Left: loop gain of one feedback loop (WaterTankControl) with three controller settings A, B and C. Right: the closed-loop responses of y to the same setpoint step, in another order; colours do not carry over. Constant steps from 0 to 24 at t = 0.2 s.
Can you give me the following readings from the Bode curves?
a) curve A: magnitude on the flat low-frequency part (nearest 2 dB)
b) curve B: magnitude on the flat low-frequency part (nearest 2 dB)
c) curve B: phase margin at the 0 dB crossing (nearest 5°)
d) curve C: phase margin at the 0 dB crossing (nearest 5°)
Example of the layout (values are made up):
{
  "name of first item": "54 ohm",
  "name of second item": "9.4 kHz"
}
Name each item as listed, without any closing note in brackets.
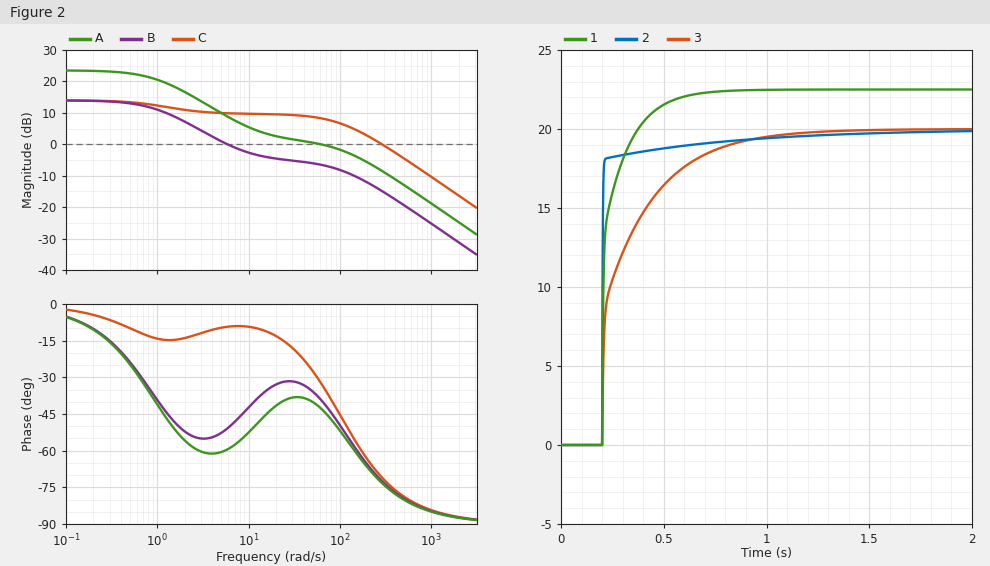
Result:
{
  "curve A: magnitude on the flat low-frequency part": "24 dB",
  "curve B: magnitude on the flat low-frequency part": "14 dB",
  "curve B: phase margin at the 0 dB crossing": "130°",
  "curve C: phase margin at the 0 dB crossing": "110°"
}
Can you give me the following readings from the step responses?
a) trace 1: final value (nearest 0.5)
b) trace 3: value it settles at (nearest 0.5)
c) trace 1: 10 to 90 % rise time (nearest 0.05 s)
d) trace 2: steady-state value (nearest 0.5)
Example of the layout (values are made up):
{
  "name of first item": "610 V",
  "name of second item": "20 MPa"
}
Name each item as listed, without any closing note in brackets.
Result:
{
  "trace 1: final value": "22.5",
  "trace 3: value it settles at": "20.0",
  "trace 1: 10 to 90 % rise time": "0.20 s",
  "trace 2: steady-state value": "20.0"
}
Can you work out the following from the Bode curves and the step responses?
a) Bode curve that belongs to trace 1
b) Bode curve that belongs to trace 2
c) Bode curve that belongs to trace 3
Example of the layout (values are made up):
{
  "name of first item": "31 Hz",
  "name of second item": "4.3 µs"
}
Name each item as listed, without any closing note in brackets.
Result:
{
  "Bode curve that belongs to trace 1": "A",
  "Bode curve that belongs to trace 2": "C",
  "Bode curve that belongs to trace 3": "B"
}
